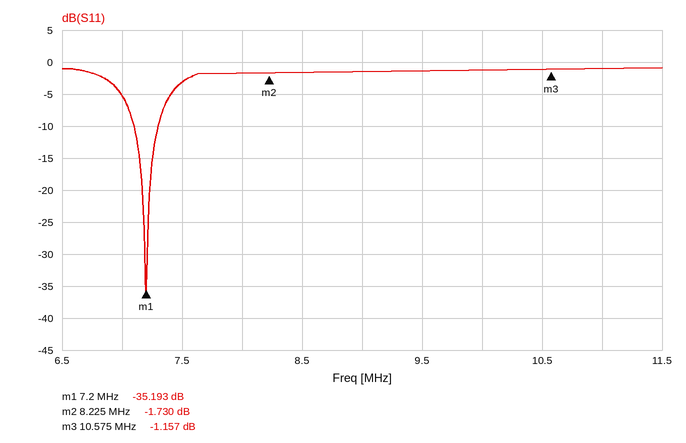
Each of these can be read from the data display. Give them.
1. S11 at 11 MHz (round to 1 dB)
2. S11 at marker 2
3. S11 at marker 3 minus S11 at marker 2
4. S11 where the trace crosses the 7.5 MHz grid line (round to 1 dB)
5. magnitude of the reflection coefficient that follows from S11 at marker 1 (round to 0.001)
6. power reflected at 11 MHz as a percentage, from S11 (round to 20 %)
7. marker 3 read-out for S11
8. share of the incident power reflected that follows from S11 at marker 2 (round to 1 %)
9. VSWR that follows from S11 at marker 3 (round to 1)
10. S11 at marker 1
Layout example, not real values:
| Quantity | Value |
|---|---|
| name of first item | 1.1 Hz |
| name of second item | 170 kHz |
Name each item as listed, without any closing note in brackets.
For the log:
| Quantity | Value |
|---|---|
| S11 at 11 MHz | -1 dB |
| S11 at marker 2 | -1.730 dB |
| S11 at marker 3 minus S11 at marker 2 | 0.573 dB |
| S11 where the trace crosses the 7.5 MHz grid line | -3 dB |
| magnitude of the reflection coefficient that follows from S11 at marker 1 | 0.017 |
| power reflected at 11 MHz as a percentage, from S11 | 80 % |
| marker 3 read-out for S11 | -1.157 dB |
| share of the incident power reflected that follows from S11 at marker 2 | 67 % |
| VSWR that follows from S11 at marker 3 | 15 |
| S11 at marker 1 | -35.193 dB |
